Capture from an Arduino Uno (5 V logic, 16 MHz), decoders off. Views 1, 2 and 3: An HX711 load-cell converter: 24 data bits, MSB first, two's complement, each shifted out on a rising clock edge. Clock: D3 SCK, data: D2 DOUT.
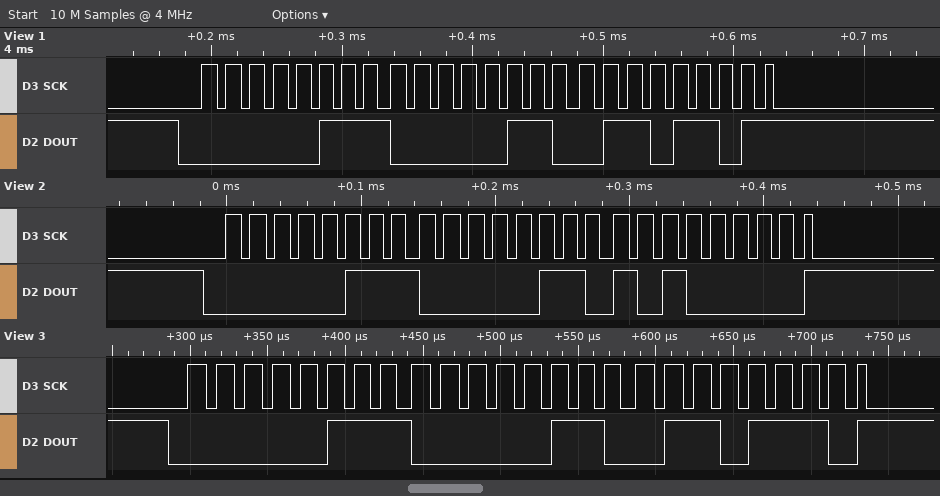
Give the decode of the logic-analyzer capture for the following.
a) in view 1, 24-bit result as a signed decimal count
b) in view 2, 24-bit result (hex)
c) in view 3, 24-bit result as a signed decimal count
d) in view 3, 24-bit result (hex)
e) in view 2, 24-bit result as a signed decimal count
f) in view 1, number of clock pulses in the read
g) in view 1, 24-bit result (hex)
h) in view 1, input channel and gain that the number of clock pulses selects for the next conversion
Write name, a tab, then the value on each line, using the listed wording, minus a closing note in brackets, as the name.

in view 1, 24-bit result as a signed decimal count	460397
in view 2, 24-bit result	0x0706A0
in view 3, 24-bit result as a signed decimal count	460398
in view 3, 24-bit result	0x07066E
in view 2, 24-bit result as a signed decimal count	460448
in view 1, number of clock pulses in the read	25
in view 1, 24-bit result	0x07066D
in view 1, input channel and gain that the number of clock pulses selects for the next conversion	channel A, gain 128
